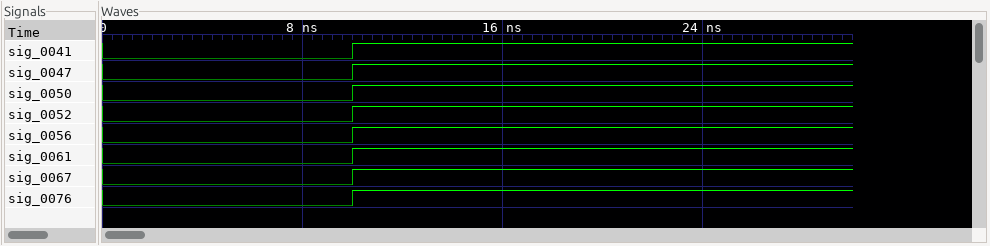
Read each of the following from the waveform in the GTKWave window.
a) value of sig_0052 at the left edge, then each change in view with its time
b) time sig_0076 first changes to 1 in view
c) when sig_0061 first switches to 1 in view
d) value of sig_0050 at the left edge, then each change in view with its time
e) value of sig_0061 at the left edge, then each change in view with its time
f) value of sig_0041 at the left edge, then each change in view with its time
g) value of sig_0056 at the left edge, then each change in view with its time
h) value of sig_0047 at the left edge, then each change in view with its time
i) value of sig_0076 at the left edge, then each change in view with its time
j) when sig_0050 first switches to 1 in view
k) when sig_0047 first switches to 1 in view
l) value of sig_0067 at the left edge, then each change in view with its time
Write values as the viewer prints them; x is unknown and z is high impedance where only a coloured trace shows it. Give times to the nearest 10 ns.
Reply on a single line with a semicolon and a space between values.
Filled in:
0, 1 at 10 ns; 10 ns; 10 ns; 0, 1 at 10 ns; 0, 1 at 10 ns; 0, 1 at 10 ns; 0, 1 at 10 ns; 0, 1 at 10 ns; 0, 1 at 10 ns; 10 ns; 10 ns; 0, 1 at 10 ns
